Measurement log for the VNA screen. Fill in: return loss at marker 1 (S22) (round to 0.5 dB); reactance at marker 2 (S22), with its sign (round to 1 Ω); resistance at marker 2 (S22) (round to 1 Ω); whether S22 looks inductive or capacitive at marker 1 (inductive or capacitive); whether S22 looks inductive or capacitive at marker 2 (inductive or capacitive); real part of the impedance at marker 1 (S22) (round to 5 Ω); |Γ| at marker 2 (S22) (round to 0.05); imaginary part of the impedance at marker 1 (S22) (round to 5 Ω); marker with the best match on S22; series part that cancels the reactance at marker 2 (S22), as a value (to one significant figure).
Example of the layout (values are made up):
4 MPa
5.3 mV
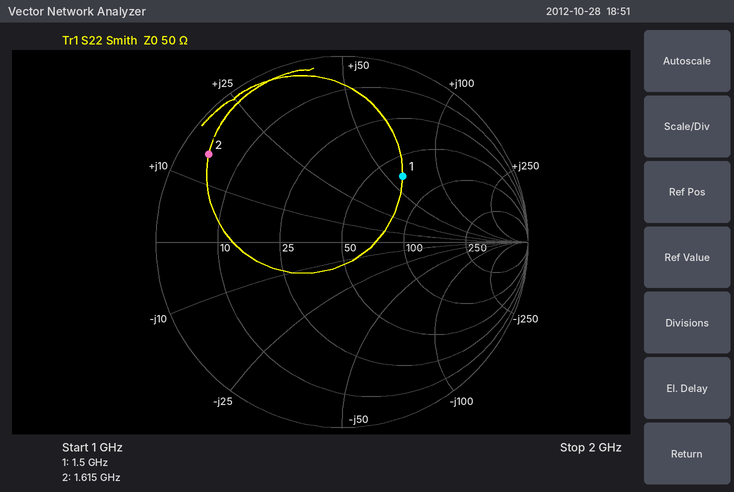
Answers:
6.5 dB
+15 Ω
4 Ω
inductive
inductive
65 Ω
0.85
+60 Ω
marker 1
7 pF
